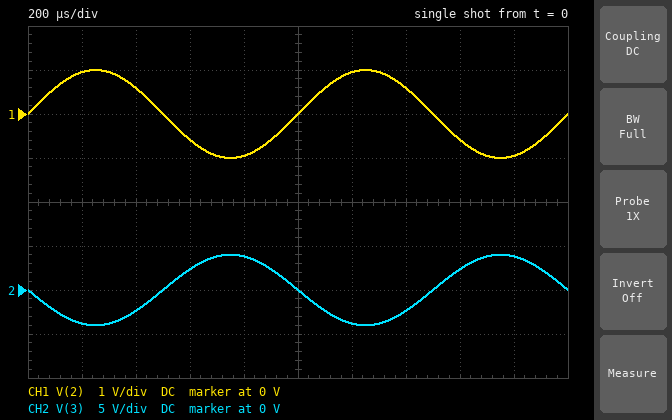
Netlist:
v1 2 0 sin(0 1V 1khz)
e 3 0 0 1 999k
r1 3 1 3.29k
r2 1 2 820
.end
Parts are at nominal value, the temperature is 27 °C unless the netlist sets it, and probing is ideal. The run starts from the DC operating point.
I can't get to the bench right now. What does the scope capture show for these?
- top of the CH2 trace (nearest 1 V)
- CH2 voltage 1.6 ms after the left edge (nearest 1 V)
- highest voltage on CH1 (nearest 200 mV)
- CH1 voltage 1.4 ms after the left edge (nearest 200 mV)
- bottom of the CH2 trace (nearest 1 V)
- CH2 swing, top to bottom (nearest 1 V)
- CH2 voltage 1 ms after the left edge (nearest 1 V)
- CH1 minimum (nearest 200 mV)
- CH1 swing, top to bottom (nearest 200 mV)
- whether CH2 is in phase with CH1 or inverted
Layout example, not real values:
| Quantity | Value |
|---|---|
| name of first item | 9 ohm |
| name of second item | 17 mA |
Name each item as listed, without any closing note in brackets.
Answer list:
| Quantity | Value |
|---|---|
| top of the CH2 trace | 4 V |
| CH2 voltage 1.6 ms after the left edge | 2 V |
| highest voltage on CH1 | 1.0 V |
| CH1 voltage 1.4 ms after the left edge | 600 mV |
| bottom of the CH2 trace | -4 V |
| CH2 swing, top to bottom | 8 V |
| CH2 voltage 1 ms after the left edge | 0 V |
| CH1 minimum | -1.0 V |
| CH1 swing, top to bottom | 2.0 V |
| whether CH2 is in phase with CH1 or inverted | inverted |
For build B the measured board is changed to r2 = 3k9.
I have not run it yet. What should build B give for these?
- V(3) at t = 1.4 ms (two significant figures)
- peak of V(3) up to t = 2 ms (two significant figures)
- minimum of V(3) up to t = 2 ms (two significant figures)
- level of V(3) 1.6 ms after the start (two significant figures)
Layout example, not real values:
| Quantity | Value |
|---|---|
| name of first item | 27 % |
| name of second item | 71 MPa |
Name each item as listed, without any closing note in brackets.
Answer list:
| Quantity | Value |
|---|---|
| V(3) at t = 1.4 ms | -500 mV |
| peak of V(3) up to t = 2 ms | 840 mV |
| minimum of V(3) up to t = 2 ms | -840 mV |
| level of V(3) 1.6 ms after the start | 500 mV |
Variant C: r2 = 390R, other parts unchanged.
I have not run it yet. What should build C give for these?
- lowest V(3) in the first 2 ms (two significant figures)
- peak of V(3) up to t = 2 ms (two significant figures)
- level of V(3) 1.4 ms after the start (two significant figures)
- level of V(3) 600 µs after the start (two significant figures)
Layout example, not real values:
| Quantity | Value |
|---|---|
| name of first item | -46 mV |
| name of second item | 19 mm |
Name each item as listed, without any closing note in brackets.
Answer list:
| Quantity | Value |
|---|---|
| lowest V(3) in the first 2 ms | -8.4 V |
| peak of V(3) up to t = 2 ms | 8.4 V |
| level of V(3) 1.4 ms after the start | -5.0 V |
| level of V(3) 600 µs after the start | 5.0 V |
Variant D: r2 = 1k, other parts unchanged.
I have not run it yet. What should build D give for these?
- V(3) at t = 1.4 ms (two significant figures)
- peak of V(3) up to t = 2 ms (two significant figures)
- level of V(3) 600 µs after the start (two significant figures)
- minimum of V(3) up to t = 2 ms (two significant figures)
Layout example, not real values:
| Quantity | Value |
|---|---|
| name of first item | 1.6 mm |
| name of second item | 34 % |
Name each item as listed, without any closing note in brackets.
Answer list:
| Quantity | Value |
|---|---|
| V(3) at t = 1.4 ms | -1.9 V |
| peak of V(3) up to t = 2 ms | 3.3 V |
| level of V(3) 600 µs after the start | 1.9 V |
| minimum of V(3) up to t = 2 ms | -3.3 V |
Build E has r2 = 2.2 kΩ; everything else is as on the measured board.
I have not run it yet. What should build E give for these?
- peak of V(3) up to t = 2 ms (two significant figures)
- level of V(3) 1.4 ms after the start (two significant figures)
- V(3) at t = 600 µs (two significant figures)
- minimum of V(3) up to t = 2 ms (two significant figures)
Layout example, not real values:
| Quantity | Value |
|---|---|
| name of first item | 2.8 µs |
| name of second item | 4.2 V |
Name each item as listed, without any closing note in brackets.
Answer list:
| Quantity | Value |
|---|---|
| peak of V(3) up to t = 2 ms | 1.5 V |
| level of V(3) 1.4 ms after the start | -880 mV |
| V(3) at t = 600 µs | 880 mV |
| minimum of V(3) up to t = 2 ms | -1.5 V |
